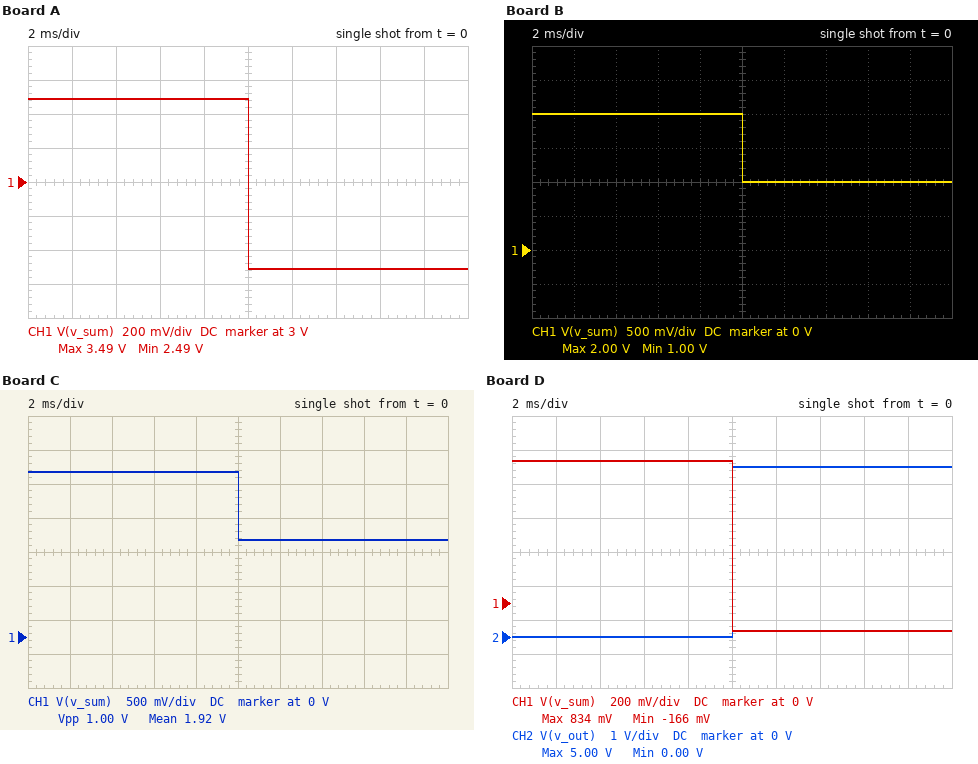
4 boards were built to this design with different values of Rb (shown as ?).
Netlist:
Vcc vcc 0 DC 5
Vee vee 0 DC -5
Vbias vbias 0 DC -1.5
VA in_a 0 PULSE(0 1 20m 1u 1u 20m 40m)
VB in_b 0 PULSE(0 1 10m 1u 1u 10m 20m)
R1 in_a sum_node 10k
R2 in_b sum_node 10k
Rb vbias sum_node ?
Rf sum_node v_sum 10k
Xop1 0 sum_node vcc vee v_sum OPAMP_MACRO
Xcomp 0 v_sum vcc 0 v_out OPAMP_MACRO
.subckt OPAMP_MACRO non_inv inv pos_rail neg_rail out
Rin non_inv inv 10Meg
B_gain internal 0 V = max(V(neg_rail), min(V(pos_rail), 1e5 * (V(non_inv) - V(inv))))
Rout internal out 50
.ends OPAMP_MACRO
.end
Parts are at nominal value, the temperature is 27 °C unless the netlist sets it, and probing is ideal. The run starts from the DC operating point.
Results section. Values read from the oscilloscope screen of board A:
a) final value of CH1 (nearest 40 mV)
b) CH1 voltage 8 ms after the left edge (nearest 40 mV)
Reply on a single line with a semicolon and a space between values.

2.48 V; 3.48 V
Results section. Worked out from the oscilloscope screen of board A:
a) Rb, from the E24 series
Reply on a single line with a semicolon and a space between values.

4.3 kΩ
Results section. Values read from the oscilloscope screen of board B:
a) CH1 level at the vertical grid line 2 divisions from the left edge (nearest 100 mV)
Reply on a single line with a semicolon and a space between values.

2.0 V
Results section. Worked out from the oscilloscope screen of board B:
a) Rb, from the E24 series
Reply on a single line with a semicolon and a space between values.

7.5 kΩ
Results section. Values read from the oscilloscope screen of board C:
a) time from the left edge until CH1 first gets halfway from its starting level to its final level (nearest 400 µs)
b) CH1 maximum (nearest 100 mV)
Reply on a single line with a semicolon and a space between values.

10.0 ms; 2.4 V
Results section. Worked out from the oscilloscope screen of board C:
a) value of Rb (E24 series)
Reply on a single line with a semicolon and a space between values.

6.2 kΩ
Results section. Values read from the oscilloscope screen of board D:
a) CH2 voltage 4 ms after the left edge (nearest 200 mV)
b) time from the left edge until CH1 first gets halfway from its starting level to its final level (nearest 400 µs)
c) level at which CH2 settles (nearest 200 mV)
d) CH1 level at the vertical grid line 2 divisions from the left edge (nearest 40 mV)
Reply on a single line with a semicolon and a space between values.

0 V; 10.0 ms; 5.0 V; 840 mV
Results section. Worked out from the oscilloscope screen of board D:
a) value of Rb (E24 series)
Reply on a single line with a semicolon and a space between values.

18 kΩ
